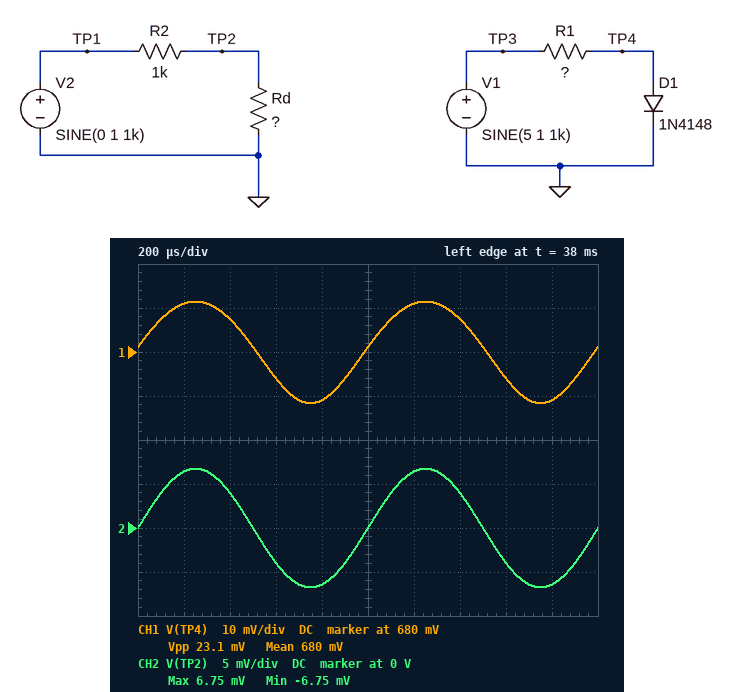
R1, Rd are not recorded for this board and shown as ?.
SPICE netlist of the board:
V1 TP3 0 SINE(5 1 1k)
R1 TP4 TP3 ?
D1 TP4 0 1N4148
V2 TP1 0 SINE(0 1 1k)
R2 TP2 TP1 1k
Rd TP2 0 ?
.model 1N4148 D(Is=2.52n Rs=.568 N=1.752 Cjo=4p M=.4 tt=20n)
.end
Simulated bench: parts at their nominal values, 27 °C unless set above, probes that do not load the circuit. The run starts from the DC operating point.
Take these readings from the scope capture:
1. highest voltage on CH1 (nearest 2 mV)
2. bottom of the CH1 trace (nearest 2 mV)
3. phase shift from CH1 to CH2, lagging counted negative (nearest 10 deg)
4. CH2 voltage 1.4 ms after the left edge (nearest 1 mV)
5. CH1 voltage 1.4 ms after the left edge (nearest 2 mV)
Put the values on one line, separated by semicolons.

692 mV; 668 mV; 0 deg; 4 mV; 688 mV
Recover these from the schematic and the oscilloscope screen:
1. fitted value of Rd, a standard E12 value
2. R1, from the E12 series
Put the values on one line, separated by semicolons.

6.8 Ω; 560 Ω
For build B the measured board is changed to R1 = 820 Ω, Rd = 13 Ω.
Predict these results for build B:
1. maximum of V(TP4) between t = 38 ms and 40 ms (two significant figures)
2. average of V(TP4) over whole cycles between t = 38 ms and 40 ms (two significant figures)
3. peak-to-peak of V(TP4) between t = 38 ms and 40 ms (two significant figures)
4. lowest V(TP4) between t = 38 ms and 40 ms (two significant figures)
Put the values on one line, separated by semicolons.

670 mV; 660 mV; 22 mV; 650 mV
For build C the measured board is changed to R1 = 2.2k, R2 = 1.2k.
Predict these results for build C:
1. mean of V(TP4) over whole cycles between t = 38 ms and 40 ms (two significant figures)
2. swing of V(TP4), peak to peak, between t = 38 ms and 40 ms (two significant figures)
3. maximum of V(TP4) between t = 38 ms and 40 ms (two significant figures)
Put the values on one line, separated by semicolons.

620 mV; 21 mV; 630 mV
